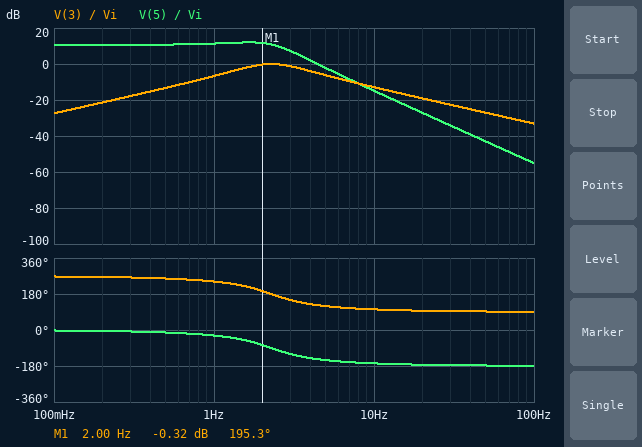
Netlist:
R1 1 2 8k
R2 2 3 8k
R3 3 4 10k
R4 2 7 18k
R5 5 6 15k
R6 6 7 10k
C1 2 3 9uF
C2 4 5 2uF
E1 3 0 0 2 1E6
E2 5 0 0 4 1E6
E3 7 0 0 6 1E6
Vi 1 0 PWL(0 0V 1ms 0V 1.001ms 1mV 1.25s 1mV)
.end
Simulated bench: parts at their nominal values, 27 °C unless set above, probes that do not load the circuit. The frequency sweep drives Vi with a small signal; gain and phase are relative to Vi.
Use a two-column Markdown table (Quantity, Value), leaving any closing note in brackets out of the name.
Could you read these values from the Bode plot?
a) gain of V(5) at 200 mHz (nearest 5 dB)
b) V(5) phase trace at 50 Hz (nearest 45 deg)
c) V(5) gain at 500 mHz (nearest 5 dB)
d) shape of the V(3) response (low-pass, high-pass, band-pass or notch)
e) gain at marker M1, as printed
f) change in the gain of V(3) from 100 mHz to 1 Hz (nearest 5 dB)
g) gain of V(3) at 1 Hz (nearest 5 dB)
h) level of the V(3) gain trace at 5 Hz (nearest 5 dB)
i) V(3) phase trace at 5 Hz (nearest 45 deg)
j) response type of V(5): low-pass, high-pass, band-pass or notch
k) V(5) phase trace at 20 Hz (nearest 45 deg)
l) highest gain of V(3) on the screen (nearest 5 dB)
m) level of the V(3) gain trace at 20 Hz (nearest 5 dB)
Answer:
| Quantity | Value |
|---|---|
| gain of V(5) at 200 mHz | 10 dB |
| V(5) phase trace at 50 Hz | -180 deg |
| V(5) gain at 500 mHz | 10 dB |
| shape of the V(3) response | band-pass |
| gain at marker M1, as printed | -0.32 dB |
| change in the gain of V(3) from 100 mHz to 1 Hz | 20 dB |
| gain of V(3) at 1 Hz | -5 dB |
| level of the V(3) gain trace at 5 Hz | -5 dB |
| V(3) phase trace at 5 Hz | 135 deg |
| response type of V(5): low-pass, high-pass, band-pass or notch | low-pass |
| V(5) phase trace at 20 Hz | -180 deg |
| highest gain of V(3) on the screen | 0 dB |
| level of the V(3) gain trace at 20 Hz | -20 dB |
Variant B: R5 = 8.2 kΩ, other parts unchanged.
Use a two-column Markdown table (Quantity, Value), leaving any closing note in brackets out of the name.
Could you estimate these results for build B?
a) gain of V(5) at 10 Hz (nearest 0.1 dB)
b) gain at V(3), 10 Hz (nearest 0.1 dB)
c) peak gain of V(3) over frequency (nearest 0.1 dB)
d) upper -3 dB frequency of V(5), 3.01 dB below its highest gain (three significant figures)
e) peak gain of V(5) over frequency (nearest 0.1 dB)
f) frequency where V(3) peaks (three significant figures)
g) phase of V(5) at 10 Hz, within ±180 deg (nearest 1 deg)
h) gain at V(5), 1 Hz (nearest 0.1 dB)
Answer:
| Quantity | Value |
|---|---|
| gain of V(5) at 10 Hz | -14.5 dB |
| gain at V(3), 10 Hz | -12.5 dB |
| peak gain of V(3) over frequency | 0 dB |
| upper -3 dB frequency of V(5), 3.01 dB below its highest gain | 3.67 Hz |
| peak gain of V(5) over frequency | 8.8 dB |
| frequency where V(3) peaks | 3.09 Hz |
| phase of V(5) at 10 Hz, within ±180 deg | -166 deg |
| gain at V(5), 1 Hz | 6.0 dB |
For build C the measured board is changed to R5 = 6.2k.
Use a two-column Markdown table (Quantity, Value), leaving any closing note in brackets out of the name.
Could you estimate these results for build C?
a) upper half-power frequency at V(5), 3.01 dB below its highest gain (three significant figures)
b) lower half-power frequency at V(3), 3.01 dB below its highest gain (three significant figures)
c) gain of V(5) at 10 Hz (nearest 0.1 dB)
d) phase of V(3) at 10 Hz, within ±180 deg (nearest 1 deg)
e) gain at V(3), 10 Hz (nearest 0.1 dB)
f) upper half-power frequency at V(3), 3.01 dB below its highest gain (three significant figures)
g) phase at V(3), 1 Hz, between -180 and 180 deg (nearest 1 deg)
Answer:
| Quantity | Value |
|---|---|
| upper half-power frequency at V(5), 3.01 dB below its highest gain | 4.20 Hz |
| lower half-power frequency at V(3), 3.01 dB below its highest gain | 2.61 Hz |
| gain of V(5) at 10 Hz | -14.2 dB |
| phase of V(3) at 10 Hz, within ±180 deg | 104 deg |
| gain at V(3), 10 Hz | -12.2 dB |
| upper half-power frequency at V(3), 3.01 dB below its highest gain | 4.82 Hz |
| phase at V(3), 1 Hz, between -180 and 180 deg | -101 deg |
